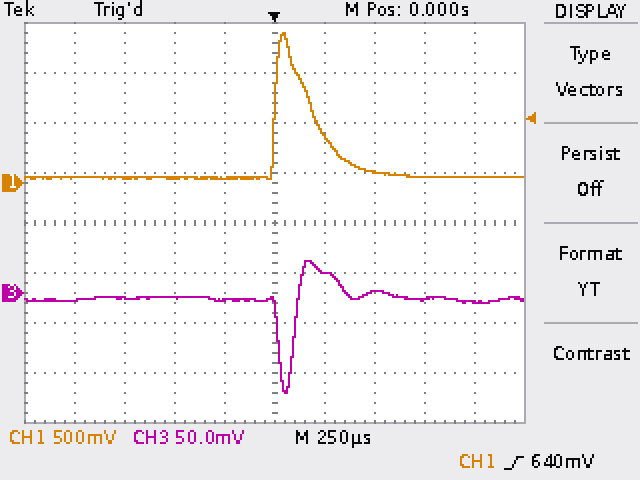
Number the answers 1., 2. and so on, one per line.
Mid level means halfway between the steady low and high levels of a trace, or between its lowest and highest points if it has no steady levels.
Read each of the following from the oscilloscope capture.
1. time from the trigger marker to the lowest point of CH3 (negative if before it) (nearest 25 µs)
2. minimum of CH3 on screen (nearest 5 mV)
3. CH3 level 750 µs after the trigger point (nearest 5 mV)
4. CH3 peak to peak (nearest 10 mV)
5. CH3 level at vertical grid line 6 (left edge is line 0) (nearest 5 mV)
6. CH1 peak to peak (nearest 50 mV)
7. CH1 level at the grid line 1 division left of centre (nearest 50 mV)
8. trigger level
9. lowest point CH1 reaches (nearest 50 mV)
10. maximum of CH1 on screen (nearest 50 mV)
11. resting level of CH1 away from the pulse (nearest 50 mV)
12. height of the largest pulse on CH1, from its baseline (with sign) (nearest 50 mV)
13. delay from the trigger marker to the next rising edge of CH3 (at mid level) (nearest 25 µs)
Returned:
1. +50 µs
2. -100 mV
3. -5 mV
4. 130 mV
5. 20 mV
6. 1.45 V
7. 50 mV
8. 640 mV
9. 50 mV
10. 1.50 V
11. 50 mV
12. +1.45 V
13. 100 µs
